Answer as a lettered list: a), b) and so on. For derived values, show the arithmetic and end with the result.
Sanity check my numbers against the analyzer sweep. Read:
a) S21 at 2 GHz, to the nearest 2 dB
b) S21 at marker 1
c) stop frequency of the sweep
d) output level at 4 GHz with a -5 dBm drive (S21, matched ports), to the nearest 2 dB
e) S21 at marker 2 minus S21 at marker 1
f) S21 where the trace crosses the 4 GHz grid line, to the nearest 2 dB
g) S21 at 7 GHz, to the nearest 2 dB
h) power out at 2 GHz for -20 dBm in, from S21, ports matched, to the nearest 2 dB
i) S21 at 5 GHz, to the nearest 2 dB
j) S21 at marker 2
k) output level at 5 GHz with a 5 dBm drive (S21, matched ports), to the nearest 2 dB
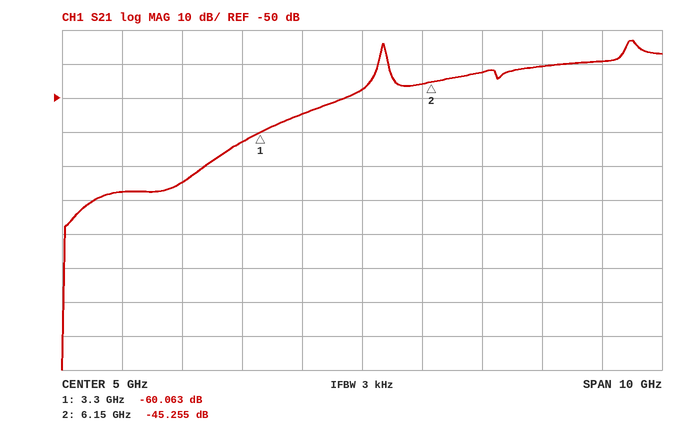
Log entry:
a) -74 dB
b) -60.063 dB
c) 10 GHz
d) -5 dBm + (-54 dB) = -60 dBm
e) -45.255 − (-60.063) = 14.808 dB
f) -54 dB
g) -42 dB
h) -20 dBm + (-74 dB) = -94 dBm
i) -48 dB
j) -45.255 dB
k) 5 dBm + (-48 dB) = -42 dBm
